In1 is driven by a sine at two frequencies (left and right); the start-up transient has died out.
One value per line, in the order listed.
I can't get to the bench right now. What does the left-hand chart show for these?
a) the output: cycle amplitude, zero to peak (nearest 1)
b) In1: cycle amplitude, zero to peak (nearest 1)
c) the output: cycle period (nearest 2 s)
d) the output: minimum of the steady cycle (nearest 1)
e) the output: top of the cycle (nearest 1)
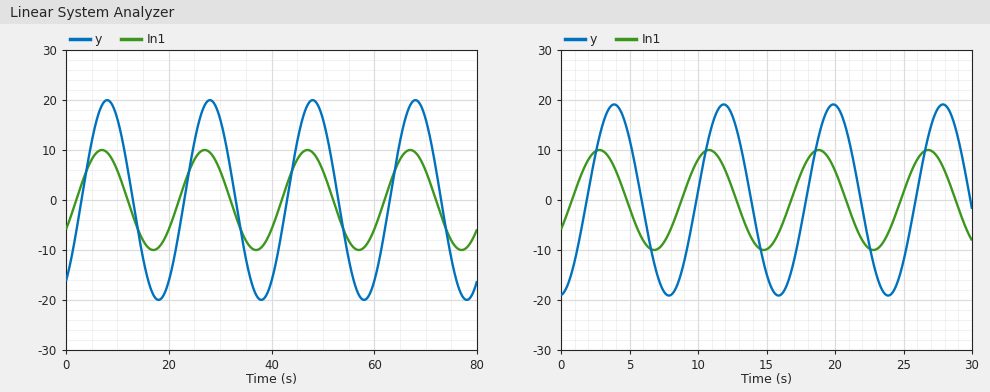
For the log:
20
10
20 s
-20
20
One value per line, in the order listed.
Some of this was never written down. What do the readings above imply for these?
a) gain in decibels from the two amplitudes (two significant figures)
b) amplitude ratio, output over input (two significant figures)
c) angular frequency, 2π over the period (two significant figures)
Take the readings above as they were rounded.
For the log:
6.0 dB
2.0
0.31 rad/s
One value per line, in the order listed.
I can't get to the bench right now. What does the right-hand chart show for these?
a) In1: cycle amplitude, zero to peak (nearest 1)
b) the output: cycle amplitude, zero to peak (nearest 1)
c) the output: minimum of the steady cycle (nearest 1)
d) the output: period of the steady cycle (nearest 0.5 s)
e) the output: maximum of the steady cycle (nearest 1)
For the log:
10
19
-19
8.0 s
19
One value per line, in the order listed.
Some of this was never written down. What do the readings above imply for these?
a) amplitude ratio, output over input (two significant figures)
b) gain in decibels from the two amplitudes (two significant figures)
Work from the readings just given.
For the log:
1.9
5.6 dB
